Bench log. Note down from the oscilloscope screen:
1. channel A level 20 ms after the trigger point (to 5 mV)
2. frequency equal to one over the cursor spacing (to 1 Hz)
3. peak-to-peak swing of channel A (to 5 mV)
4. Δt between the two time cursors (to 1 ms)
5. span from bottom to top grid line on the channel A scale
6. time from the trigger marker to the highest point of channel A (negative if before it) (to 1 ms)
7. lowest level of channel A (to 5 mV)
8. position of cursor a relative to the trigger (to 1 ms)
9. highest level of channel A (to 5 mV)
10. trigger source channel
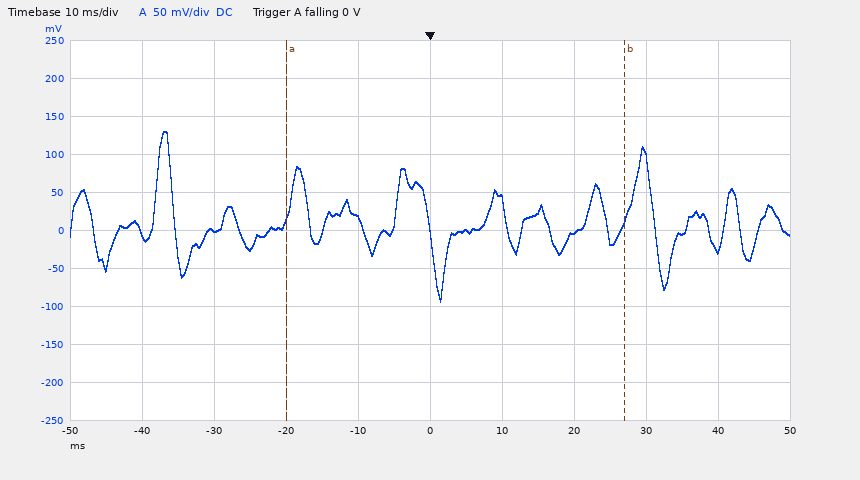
0 mV
21 Hz
225 mV
47 ms
500 mV
-37 ms
-95 mV
-20 ms
130 mV
channel A
